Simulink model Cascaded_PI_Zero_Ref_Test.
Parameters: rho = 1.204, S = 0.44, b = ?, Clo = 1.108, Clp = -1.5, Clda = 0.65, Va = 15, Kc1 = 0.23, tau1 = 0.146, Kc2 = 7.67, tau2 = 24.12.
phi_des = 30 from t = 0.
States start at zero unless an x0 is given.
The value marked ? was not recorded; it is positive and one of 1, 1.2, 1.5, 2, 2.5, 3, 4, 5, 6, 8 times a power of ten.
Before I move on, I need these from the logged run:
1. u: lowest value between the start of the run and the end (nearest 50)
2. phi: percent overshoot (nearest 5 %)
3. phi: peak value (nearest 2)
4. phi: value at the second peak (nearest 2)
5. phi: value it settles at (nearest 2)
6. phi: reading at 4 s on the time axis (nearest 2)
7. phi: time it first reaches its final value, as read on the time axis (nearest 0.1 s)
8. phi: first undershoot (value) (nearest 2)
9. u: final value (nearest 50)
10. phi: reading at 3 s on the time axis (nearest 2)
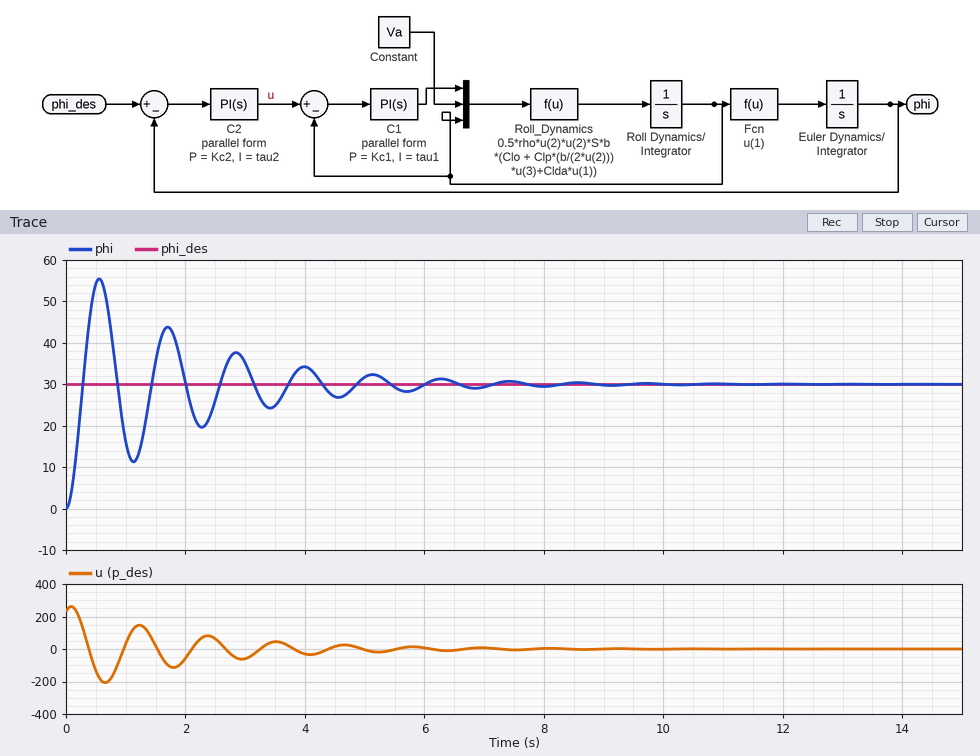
-200
85 %
56
44
30
34
0.3 s
12
0
36
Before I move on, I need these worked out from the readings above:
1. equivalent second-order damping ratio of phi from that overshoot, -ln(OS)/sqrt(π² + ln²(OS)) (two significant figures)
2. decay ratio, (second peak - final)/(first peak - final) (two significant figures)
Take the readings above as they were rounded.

0.052
0.54
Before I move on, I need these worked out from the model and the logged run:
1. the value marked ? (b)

0.5
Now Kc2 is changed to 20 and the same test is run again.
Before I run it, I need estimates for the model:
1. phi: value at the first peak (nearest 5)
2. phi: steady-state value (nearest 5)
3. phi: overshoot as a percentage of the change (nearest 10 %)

50
30
60 %
